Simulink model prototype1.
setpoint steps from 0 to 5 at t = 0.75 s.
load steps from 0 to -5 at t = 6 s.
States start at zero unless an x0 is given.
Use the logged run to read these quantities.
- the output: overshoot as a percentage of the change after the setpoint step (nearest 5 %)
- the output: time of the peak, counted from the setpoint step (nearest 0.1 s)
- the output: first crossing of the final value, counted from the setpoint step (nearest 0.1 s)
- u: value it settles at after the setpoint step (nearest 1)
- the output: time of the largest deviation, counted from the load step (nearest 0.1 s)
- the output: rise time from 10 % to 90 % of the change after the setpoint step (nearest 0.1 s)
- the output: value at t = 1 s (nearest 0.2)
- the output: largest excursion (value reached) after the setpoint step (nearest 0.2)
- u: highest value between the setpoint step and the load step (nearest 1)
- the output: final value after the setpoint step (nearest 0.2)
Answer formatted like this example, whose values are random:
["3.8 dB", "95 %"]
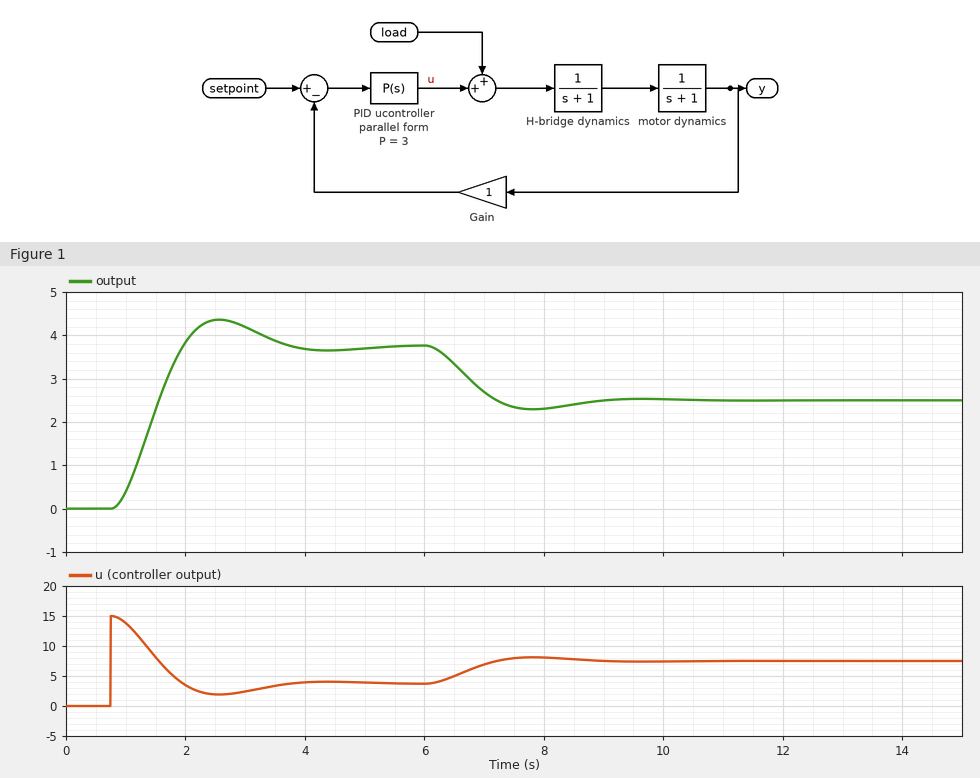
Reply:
["15 %", "1.8 s", "1.2 s", "4", "1.8 s", "0.8 s", "0.4", "4.4", "15", "3.8"]
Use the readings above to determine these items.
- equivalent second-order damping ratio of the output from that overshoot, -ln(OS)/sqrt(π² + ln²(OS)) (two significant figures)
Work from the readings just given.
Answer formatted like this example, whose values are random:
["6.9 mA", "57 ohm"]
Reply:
["0.52"]
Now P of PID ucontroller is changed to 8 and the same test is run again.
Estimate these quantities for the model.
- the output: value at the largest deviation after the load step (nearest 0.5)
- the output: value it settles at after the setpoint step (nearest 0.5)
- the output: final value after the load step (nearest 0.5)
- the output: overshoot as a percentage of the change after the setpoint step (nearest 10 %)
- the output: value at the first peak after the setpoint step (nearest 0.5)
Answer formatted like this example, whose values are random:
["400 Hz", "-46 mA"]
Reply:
["3.5", "4.5", "4.0", "30 %", "6.0"]
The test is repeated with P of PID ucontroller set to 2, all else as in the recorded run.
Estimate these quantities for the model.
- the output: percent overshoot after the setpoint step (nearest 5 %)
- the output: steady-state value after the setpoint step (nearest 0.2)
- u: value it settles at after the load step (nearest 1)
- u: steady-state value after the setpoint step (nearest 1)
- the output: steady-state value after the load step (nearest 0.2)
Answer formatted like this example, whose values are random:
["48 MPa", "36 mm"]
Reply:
["10 %", "3.4", "7", "3", "1.6"]
